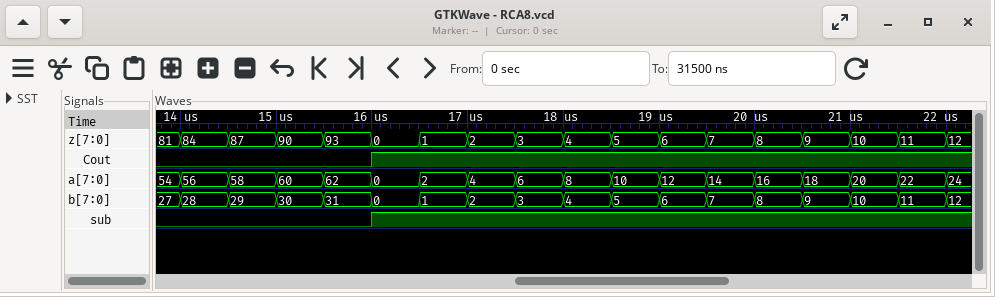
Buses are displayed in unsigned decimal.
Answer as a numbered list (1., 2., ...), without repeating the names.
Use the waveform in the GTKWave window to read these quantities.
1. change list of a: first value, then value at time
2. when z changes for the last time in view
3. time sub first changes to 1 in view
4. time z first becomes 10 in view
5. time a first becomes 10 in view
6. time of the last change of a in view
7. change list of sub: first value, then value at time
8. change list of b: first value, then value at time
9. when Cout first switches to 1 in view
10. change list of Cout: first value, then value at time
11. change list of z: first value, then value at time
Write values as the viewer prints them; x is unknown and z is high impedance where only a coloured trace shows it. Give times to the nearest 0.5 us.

1. 54, 56 at 14 us, 58 at 14.5 us, 60 at 15 us, 62 at 15.5 us, 0 at 16 us, 2 at 16.5 us, 4 at 17 us, 6 at 17.5 us, 8 at 18 us, 10 at 18.5 us, 12 at 19 us, 14 at 19.5 us, 16 at 20 us, 18 at 20.5 us, 20 at 21 us, 22 at 21.5 us, 24 at 22 us
2. 22 us
3. 16 us
4. 21 us
5. 18.5 us
6. 22 us
7. 0, 1 at 16 us
8. 27, 28 at 14 us, 29 at 14.5 us, 30 at 15 us, 31 at 15.5 us, 0 at 16 us, 1 at 16.5 us, 2 at 17 us, 3 at 17.5 us, 4 at 18 us, 5 at 18.5 us, 6 at 19 us, 7 at 19.5 us, 8 at 20 us, 9 at 20.5 us, 10 at 21 us, 11 at 21.5 us, 12 at 22 us
9. 16 us
10. 0, 1 at 16 us
11. 81, 84 at 14 us, 87 at 14.5 us, 90 at 15 us, 93 at 15.5 us, 0 at 16 us, 1 at 16.5 us, 2 at 17 us, 3 at 17.5 us, 4 at 18 us, 5 at 18.5 us, 6 at 19 us, 7 at 19.5 us, 8 at 20 us, 9 at 20.5 us, 10 at 21 us, 11 at 21.5 us, 12 at 22 us
